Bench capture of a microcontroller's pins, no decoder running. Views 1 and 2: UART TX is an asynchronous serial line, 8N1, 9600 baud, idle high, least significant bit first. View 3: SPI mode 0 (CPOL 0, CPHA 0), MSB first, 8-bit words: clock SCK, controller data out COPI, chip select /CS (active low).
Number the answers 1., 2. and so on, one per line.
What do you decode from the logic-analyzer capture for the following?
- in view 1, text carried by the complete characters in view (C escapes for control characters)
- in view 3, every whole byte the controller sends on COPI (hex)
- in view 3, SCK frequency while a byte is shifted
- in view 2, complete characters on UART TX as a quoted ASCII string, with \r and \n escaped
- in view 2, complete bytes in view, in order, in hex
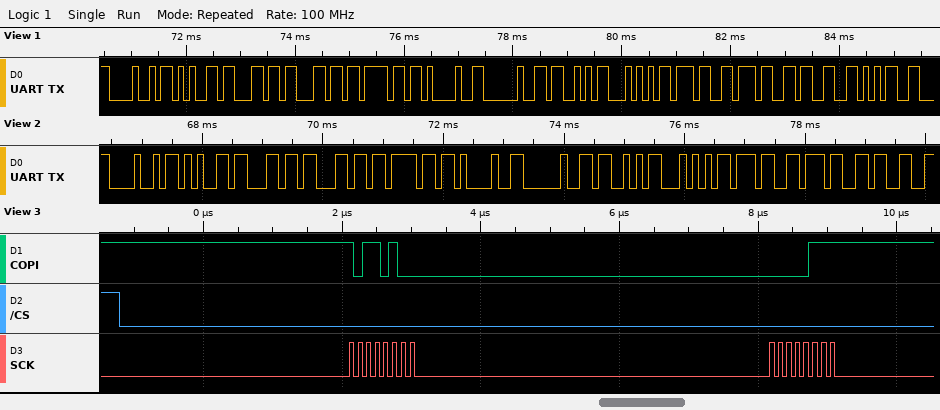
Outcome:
1. "Hello! ST7735"
2. 0xB4 0x07
3. 8 MHz
4. "Hello! ST773"
5. 48 65 6C 6C 6F 21 20 53 54 37 37 33
